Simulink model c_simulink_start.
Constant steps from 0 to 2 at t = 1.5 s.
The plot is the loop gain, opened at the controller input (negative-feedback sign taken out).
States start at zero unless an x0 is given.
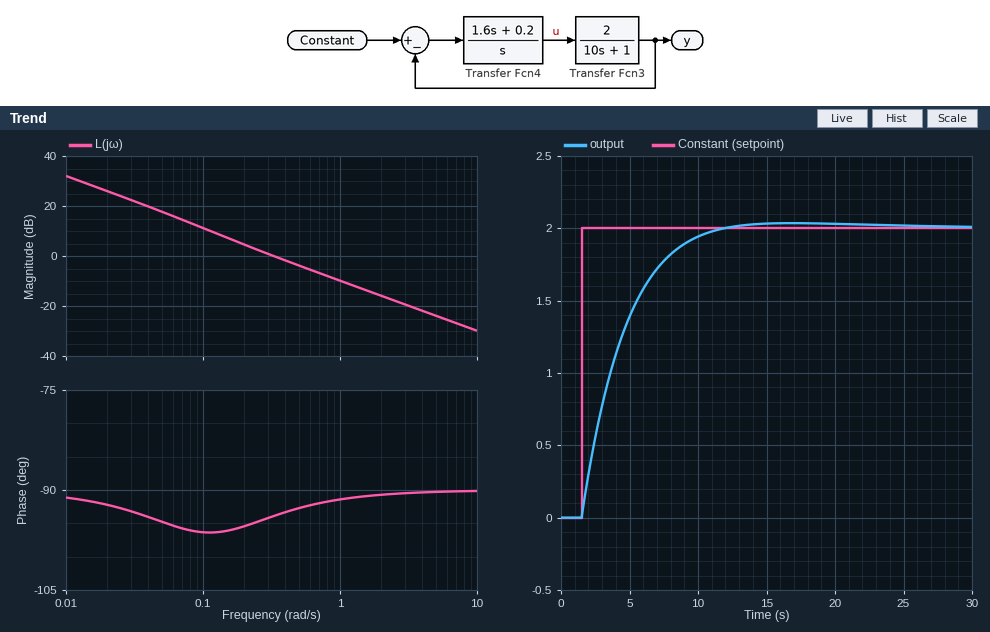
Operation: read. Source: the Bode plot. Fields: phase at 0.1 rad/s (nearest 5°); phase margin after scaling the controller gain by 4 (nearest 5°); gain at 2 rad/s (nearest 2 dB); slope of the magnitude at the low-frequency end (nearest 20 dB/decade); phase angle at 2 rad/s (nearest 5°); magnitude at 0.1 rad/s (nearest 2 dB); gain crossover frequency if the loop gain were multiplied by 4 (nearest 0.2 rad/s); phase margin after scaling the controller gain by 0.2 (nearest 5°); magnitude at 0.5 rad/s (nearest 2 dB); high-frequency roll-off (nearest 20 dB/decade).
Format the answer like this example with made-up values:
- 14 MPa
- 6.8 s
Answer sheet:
- -95°
- 90°
- -16 dB
- -20 dB/decade
- -90°
- 12 dB
- 1.2 rad/s
- 85°
- -4 dB
- -20 dB/decade
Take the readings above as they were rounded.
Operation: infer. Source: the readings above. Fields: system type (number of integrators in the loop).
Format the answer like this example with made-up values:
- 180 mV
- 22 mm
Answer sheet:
- 1
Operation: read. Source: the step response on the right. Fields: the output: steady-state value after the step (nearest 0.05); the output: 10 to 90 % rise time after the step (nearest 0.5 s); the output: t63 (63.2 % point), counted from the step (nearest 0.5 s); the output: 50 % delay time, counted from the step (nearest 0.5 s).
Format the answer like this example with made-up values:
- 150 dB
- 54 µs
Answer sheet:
- 2.00
- 6.0 s
- 3.0 s
- 2.0 s
